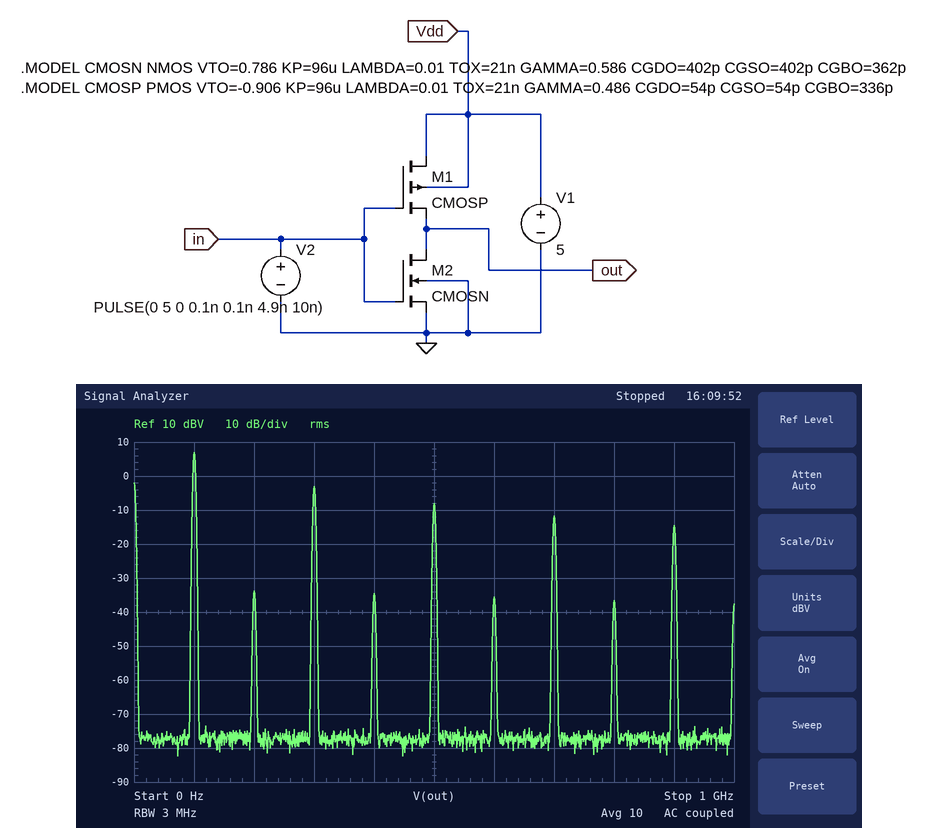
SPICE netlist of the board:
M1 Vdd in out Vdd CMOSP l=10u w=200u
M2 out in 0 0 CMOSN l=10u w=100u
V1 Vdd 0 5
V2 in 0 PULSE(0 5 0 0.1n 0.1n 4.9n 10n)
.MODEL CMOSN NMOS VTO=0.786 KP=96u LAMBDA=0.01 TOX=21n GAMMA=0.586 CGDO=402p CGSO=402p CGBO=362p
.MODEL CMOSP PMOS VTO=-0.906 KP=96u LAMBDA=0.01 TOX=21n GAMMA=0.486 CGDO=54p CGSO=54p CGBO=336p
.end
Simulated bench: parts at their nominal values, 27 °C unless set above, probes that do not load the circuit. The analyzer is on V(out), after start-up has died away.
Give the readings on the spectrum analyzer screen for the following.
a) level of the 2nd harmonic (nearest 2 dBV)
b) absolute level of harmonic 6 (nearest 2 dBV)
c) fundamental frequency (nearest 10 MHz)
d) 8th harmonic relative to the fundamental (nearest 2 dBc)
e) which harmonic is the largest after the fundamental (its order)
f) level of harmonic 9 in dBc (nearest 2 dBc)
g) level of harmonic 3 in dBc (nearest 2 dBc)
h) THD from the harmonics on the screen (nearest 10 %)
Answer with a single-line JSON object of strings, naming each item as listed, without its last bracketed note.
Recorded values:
{"level of the 2nd harmonic": "-34 dBV", "absolute level of harmonic 6": "-36 dBV", "fundamental frequency": "100 MHz", "8th harmonic relative to the fundamental": "-44 dBc", "which harmonic is the largest after the fundamental": "3", "level of harmonic 9 in dBc": "-22 dBc", "level of harmonic 3 in dBc": "-10 dBc", "THD from the harmonics on the screen": "40 %"}
